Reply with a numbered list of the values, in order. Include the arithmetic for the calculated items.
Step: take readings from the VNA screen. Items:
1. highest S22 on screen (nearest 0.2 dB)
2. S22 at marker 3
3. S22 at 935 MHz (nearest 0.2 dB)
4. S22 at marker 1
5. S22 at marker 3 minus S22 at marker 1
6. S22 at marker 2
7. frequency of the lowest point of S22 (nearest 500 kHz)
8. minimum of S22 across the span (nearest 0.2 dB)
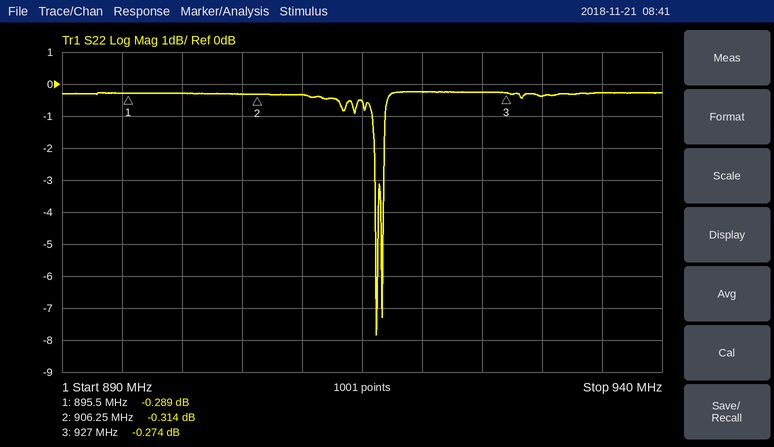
1. -0.2 dB
2. -0.274 dB
3. -0.2 dB
4. -0.289 dB
5. -0.274 − (-0.289) = 0.015 dB
6. -0.314 dB
7. 916.0 MHz
8. -7.8 dB
